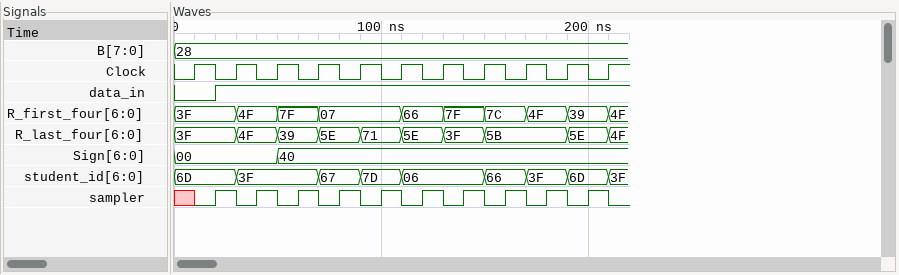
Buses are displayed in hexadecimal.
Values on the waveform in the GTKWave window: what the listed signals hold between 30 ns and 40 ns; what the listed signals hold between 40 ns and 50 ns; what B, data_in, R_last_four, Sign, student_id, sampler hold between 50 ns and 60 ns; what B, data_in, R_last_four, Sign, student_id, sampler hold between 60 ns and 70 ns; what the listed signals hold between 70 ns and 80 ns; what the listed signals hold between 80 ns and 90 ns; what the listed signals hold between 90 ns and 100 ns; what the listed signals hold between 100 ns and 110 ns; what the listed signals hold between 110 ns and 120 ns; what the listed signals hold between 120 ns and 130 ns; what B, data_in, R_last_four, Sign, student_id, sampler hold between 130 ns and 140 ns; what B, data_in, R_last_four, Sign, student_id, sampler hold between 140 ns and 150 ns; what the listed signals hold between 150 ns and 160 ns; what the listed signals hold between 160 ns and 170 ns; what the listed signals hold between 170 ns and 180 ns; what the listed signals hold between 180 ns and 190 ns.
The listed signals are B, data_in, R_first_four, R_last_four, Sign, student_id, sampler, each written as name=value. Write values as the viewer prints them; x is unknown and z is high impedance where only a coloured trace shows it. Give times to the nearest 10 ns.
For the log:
B=28, data_in=1, R_first_four=4F, R_last_four=4F, Sign=00, student_id=3F, sampler=0
B=28, data_in=1, R_first_four=4F, R_last_four=4F, Sign=00, student_id=3F, sampler=1
B=28, data_in=1, R_last_four=39, Sign=40, student_id=3F, sampler=0
B=28, data_in=1, R_last_four=39, Sign=40, student_id=3F, sampler=1
B=28, data_in=1, R_first_four=07, R_last_four=5E, Sign=40, student_id=67, sampler=0
B=28, data_in=1, R_first_four=07, R_last_four=5E, Sign=40, student_id=67, sampler=1
B=28, data_in=1, R_first_four=07, R_last_four=71, Sign=40, student_id=7D, sampler=0
B=28, data_in=1, R_first_four=07, R_last_four=71, Sign=40, student_id=7D, sampler=1
B=28, data_in=1, R_first_four=66, R_last_four=5E, Sign=40, student_id=06, sampler=0
B=28, data_in=1, R_first_four=66, R_last_four=5E, Sign=40, student_id=06, sampler=1
B=28, data_in=1, R_last_four=3F, Sign=40, student_id=06, sampler=0
B=28, data_in=1, R_last_four=3F, Sign=40, student_id=06, sampler=1
B=28, data_in=1, R_first_four=7C, R_last_four=5B, Sign=40, student_id=66, sampler=0
B=28, data_in=1, R_first_four=7C, R_last_four=5B, Sign=40, student_id=66, sampler=1
B=28, data_in=1, R_first_four=4F, R_last_four=5B, Sign=40, student_id=3F, sampler=0
B=28, data_in=1, R_first_four=4F, R_last_four=5B, Sign=40, student_id=3F, sampler=1
